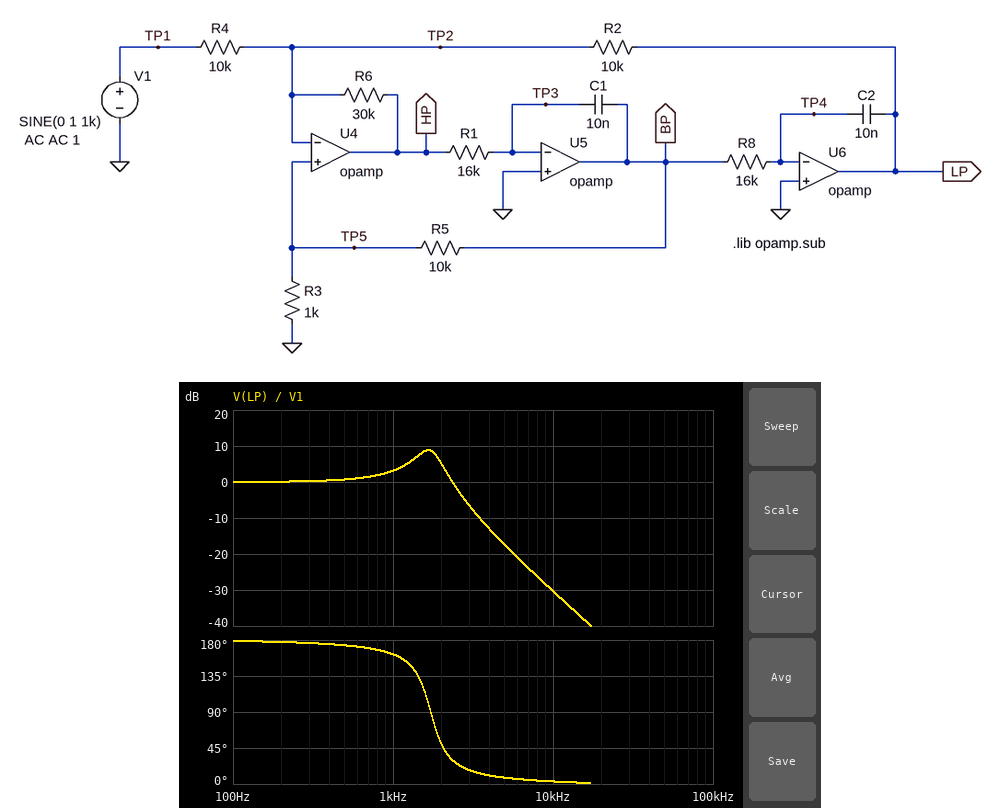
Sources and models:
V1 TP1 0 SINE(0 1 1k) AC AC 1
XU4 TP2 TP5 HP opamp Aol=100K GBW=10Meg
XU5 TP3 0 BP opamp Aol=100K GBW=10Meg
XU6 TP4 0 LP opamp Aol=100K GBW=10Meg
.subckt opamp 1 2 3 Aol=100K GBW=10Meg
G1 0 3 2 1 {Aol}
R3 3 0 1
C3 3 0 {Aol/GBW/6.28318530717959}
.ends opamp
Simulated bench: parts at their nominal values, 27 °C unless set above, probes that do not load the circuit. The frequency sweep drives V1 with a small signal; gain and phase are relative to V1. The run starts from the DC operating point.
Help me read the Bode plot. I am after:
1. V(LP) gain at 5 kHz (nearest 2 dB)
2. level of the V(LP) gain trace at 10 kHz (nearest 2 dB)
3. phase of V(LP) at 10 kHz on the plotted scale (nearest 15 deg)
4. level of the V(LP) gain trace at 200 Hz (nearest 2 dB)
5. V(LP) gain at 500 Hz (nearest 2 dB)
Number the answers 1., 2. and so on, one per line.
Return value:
1. -18 dB
2. -30 dB
3. 0 deg
4. 0 dB
5. 0 dB
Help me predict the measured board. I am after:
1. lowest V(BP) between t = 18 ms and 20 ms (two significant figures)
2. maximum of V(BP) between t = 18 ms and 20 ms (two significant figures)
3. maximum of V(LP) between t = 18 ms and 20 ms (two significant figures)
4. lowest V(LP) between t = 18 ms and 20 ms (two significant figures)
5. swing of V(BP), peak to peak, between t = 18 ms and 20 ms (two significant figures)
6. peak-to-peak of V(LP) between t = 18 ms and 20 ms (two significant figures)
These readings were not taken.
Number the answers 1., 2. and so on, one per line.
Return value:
1. -1.4 V
2. 1.4 V
3. 1.4 V
4. -1.4 V
5. 2.9 V
6. 2.9 V
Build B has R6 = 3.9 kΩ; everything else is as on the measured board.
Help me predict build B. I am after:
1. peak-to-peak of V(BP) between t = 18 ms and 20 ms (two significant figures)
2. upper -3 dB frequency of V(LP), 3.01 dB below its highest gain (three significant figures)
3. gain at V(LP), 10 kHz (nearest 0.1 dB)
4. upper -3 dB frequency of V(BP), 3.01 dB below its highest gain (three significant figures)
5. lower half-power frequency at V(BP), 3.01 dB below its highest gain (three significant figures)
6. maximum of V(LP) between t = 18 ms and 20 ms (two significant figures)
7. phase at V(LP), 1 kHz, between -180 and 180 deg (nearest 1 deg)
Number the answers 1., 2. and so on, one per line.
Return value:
1. 1.2 V
2. 687 Hz
3. -48.2 dB
4. 707 Hz
5. 546 Hz
6. 610 mV
7. 15 deg
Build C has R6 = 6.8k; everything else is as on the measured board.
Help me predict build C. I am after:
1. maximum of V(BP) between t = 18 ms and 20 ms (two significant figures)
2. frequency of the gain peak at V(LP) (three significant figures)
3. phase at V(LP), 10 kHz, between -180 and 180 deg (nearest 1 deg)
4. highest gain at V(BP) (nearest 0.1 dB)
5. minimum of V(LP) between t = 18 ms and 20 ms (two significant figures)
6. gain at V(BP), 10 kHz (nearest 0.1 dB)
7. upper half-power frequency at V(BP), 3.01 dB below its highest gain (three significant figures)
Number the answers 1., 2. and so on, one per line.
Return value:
1. 1.7 V
2. 806 Hz
3. 1 deg
4. 10.0 dB
5. -1.7 V
6. -23.3 dB
7. 934 Hz
